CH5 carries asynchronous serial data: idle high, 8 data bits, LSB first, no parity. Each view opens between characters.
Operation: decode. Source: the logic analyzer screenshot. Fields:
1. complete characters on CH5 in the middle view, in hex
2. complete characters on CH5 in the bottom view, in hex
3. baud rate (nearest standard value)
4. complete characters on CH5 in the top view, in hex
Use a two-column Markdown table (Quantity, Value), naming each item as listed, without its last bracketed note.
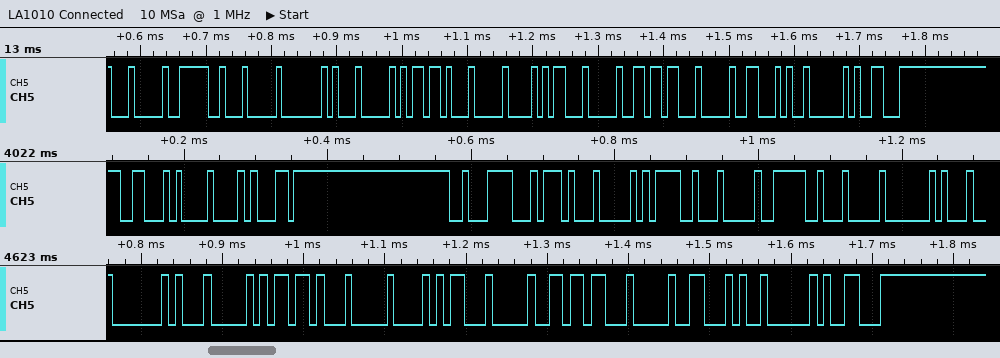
| Quantity | Value |
|---|---|
| complete characters on CH5 in the middle view, in hex | 46, 08, B1, E2, 74, 04, 3D, 04, 3E, 04, 40 |
| complete characters on CH5 in the bottom view, in hex | 40, 04, 6D, 04, A8, 04, B6, 04, 46, 02, 19 |
| baud rate | 115200 baud |
| complete characters on CH5 in the top view, in hex | 04, 3E, 04, 40, 04, 6D, 04, A8, 04, B6, 04, 46, 02, 19 |
